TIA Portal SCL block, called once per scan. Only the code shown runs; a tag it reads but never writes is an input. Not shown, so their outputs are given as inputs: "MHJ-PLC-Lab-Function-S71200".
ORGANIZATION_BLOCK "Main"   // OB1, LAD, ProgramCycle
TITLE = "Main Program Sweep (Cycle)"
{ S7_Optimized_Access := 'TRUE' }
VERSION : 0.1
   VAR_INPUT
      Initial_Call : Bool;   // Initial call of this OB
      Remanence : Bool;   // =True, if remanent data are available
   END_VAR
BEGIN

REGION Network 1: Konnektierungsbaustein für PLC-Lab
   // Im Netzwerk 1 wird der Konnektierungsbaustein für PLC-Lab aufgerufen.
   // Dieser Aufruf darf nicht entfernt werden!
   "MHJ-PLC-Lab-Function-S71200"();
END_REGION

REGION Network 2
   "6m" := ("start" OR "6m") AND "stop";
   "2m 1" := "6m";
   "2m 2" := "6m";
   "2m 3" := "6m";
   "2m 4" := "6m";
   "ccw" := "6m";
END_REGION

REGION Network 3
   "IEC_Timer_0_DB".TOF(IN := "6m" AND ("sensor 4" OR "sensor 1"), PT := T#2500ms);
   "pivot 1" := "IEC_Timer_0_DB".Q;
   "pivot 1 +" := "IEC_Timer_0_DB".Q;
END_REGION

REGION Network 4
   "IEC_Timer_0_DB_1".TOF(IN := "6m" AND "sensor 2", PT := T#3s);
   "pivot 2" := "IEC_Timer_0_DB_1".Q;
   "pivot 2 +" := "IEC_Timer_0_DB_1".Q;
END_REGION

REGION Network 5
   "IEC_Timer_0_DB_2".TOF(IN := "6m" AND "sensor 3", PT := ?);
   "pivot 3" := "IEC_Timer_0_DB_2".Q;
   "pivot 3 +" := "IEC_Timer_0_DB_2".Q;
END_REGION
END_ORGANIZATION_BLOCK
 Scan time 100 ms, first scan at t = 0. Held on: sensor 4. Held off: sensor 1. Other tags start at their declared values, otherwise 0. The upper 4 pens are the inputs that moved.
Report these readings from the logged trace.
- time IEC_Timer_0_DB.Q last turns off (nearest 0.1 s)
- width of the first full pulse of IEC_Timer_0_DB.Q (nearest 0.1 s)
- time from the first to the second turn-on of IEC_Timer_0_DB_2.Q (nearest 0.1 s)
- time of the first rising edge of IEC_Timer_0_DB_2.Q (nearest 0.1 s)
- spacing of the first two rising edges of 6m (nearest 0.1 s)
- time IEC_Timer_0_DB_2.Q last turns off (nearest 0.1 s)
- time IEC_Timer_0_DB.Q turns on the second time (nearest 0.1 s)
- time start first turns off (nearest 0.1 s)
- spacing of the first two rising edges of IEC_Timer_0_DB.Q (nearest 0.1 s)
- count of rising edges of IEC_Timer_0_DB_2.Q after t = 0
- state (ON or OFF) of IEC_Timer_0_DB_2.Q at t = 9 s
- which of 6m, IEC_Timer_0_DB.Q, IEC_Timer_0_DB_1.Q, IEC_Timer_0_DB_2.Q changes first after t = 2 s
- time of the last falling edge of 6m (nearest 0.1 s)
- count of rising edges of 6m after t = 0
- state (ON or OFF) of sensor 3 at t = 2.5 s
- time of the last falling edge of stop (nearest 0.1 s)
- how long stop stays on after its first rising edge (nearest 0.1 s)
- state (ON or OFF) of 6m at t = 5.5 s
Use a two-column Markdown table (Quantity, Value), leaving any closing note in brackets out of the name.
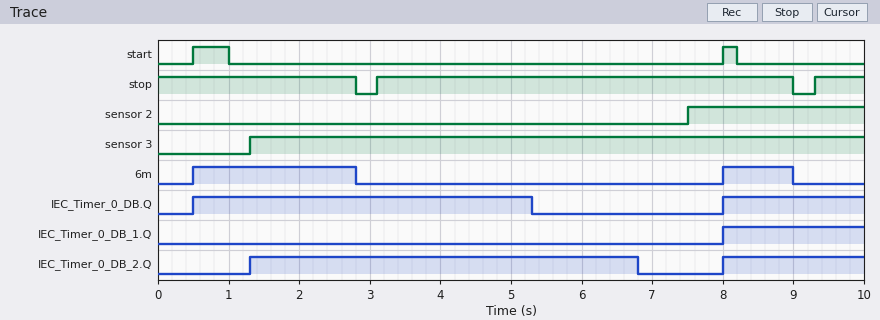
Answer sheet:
| Quantity | Value |
|---|---|
| time IEC_Timer_0_DB.Q last turns off | 5.3 s |
| width of the first full pulse of IEC_Timer_0_DB.Q | 4.8 s |
| time from the first to the second turn-on of IEC_Timer_0_DB_2.Q | 6.7 s |
| time of the first rising edge of IEC_Timer_0_DB_2.Q | 1.3 s |
| spacing of the first two rising edges of 6m | 7.5 s |
| time IEC_Timer_0_DB_2.Q last turns off | 6.8 s |
| time IEC_Timer_0_DB.Q turns on the second time | 8.0 s |
| time start first turns off | 1.0 s |
| spacing of the first two rising edges of IEC_Timer_0_DB.Q | 7.5 s |
| count of rising edges of IEC_Timer_0_DB_2.Q after t = 0 | 2 |
| state (ON or OFF) of IEC_Timer_0_DB_2.Q at t = 9 s | ON |
| which of 6m, IEC_Timer_0_DB.Q, IEC_Timer_0_DB_1.Q, IEC_Timer_0_DB_2.Q changes first after t = 2 s | 6m |
| time of the last falling edge of 6m | 9.0 s |
| count of rising edges of 6m after t = 0 | 2 |
| state (ON or OFF) of sensor 3 at t = 2.5 s | ON |
| time of the last falling edge of stop | 9.0 s |
| how long stop stays on after its first rising edge | 5.9 s |
| state (ON or OFF) of 6m at t = 5.5 s | OFF |
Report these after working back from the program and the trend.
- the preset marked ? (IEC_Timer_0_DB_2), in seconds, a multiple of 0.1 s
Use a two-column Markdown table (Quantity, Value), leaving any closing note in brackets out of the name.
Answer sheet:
| Quantity | Value |
|---|---|
| the preset marked ? (IEC_Timer_0_DB_2), in seconds, a multiple of 0.1 s | 4.0 s |
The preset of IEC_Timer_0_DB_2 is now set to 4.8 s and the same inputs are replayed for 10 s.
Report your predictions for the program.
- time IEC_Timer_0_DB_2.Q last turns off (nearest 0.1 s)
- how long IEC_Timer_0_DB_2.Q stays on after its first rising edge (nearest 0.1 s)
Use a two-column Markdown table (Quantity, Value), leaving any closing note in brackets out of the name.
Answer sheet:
| Quantity | Value |
|---|---|
| time IEC_Timer_0_DB_2.Q last turns off | 7.6 s |
| how long IEC_Timer_0_DB_2.Q stays on after its first rising edge | 6.3 s |
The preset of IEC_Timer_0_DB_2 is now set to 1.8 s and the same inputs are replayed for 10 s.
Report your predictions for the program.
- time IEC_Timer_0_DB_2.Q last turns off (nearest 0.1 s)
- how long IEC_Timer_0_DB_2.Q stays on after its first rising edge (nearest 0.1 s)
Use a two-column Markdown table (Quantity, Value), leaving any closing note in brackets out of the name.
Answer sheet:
| Quantity | Value |
|---|---|
| time IEC_Timer_0_DB_2.Q last turns off | 4.6 s |
| how long IEC_Timer_0_DB_2.Q stays on after its first rising edge | 3.3 s |
